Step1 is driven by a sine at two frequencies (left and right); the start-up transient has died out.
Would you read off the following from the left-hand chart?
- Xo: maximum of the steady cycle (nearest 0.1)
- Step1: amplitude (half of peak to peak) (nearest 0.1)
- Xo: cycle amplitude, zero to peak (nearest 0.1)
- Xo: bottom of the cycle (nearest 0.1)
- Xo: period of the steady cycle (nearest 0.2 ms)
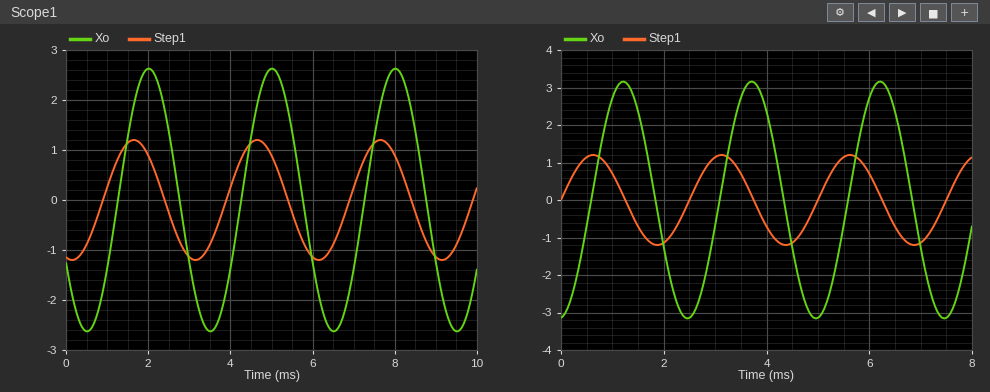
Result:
2.6
1.2
2.6
-2.6
3.0 ms
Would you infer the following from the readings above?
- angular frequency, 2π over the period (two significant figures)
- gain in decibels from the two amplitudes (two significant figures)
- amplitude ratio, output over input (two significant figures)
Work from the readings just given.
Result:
2.1 rad/ms
6.7 dB
2.2
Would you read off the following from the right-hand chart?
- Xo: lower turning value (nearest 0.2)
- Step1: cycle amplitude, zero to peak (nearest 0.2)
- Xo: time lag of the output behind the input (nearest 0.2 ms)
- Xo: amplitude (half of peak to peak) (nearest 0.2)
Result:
-3.2
1.2
0.6 ms
3.2
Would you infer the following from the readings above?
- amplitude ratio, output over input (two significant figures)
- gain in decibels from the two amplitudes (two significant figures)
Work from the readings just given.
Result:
2.7
8.5 dB
